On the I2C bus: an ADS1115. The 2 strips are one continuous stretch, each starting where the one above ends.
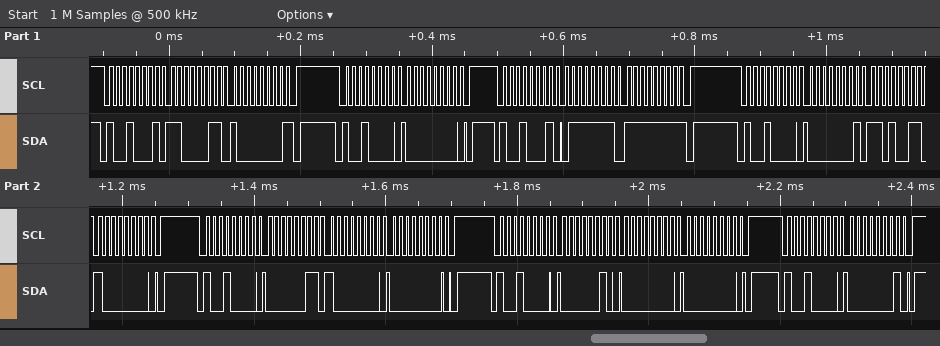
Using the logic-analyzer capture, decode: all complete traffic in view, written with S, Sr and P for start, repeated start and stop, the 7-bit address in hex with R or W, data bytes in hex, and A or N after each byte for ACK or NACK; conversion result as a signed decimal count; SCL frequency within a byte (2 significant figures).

S 48R A C3 A 80 N P S 48W A 00 A P S 48R A 7F A FF N P S 48W A 01 A D3 A 80 A P S 48W A 03 A 80 A 00 A P S 48W A 02 A 00 A 00 A P S 48W A 01 A P
32767
100 kHz
